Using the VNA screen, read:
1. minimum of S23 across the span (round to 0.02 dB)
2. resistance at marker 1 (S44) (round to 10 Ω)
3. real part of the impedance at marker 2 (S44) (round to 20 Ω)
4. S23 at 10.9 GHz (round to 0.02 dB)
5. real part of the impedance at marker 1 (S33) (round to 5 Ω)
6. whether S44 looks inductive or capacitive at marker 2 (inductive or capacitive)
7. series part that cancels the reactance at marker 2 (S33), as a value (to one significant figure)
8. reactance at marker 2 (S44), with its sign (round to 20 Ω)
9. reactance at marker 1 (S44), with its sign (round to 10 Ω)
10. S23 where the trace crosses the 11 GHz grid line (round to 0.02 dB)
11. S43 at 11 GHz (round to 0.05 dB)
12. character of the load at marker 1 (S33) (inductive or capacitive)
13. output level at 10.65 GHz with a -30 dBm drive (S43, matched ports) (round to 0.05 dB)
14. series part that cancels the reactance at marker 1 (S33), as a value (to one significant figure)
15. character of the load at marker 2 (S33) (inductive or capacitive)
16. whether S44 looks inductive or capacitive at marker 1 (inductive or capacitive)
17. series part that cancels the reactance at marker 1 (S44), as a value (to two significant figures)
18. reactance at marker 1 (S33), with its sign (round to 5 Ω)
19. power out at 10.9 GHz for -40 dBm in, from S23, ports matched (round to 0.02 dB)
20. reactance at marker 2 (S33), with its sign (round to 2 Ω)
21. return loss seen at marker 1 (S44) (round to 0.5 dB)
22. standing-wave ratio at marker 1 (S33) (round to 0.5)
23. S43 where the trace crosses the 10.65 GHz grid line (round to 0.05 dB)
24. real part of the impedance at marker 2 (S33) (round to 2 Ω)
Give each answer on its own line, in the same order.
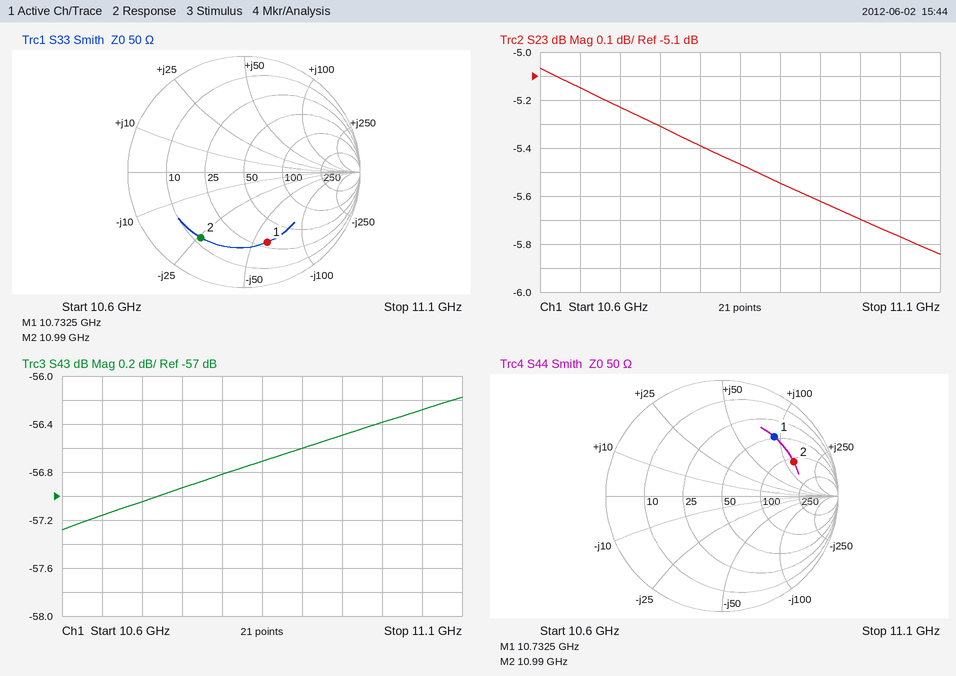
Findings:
-5.84 dB
50 Ω
120 Ω
-5.54 dB
30 Ω
inductive
400 pH
+120 Ω
+90 Ω
-5.70 dB
-56.40 dB
capacitive
-87.15 dBm
900 pH
capacitive
inductive
160 fF
-60 Ω
-45.54 dBm
-26 Ω
3.5 dB
4.5
-57.15 dB
12 Ω
